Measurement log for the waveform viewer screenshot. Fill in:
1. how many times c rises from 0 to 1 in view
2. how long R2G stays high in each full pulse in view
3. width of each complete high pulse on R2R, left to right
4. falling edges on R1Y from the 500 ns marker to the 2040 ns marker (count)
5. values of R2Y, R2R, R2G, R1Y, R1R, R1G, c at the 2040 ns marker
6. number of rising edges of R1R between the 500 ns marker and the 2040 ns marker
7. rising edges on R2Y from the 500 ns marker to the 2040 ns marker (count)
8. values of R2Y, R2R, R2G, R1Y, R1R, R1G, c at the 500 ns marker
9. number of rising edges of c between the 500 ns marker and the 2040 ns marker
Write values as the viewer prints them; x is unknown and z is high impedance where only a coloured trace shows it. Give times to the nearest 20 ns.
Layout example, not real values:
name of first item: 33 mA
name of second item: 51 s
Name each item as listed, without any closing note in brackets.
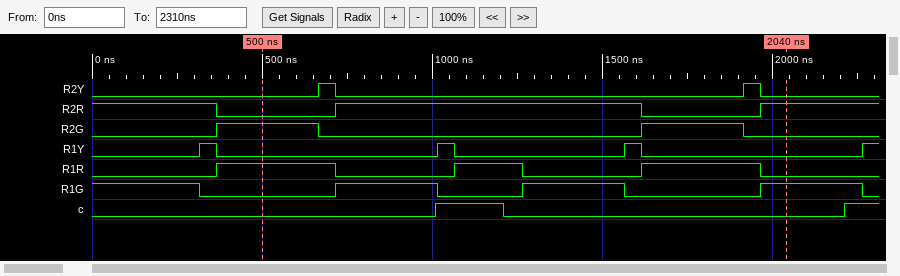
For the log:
how many times c rises from 0 to 1 in view: 2
how long R2G stays high in each full pulse in view: 300 ns, 300 ns
width of each complete high pulse on R2R, left to right: 900 ns
falling edges on R1Y from the 500 ns marker to the 2040 ns marker: 2
values of R2Y, R2R, R2G, R1Y, R1R, R1G, c at the 2040 ns marker: R2Y=0, R2R=1, R2G=0, R1Y=0, R1R=0, R1G=1, c=0
number of rising edges of R1R between the 500 ns marker and the 2040 ns marker: 2
rising edges on R2Y from the 500 ns marker to the 2040 ns marker: 2
values of R2Y, R2R, R2G, R1Y, R1R, R1G, c at the 500 ns marker: R2Y=0, R2R=0, R2G=1, R1Y=0, R1R=1, R1G=0, c=0
number of rising edges of c between the 500 ns marker and the 2040 ns marker: 1
